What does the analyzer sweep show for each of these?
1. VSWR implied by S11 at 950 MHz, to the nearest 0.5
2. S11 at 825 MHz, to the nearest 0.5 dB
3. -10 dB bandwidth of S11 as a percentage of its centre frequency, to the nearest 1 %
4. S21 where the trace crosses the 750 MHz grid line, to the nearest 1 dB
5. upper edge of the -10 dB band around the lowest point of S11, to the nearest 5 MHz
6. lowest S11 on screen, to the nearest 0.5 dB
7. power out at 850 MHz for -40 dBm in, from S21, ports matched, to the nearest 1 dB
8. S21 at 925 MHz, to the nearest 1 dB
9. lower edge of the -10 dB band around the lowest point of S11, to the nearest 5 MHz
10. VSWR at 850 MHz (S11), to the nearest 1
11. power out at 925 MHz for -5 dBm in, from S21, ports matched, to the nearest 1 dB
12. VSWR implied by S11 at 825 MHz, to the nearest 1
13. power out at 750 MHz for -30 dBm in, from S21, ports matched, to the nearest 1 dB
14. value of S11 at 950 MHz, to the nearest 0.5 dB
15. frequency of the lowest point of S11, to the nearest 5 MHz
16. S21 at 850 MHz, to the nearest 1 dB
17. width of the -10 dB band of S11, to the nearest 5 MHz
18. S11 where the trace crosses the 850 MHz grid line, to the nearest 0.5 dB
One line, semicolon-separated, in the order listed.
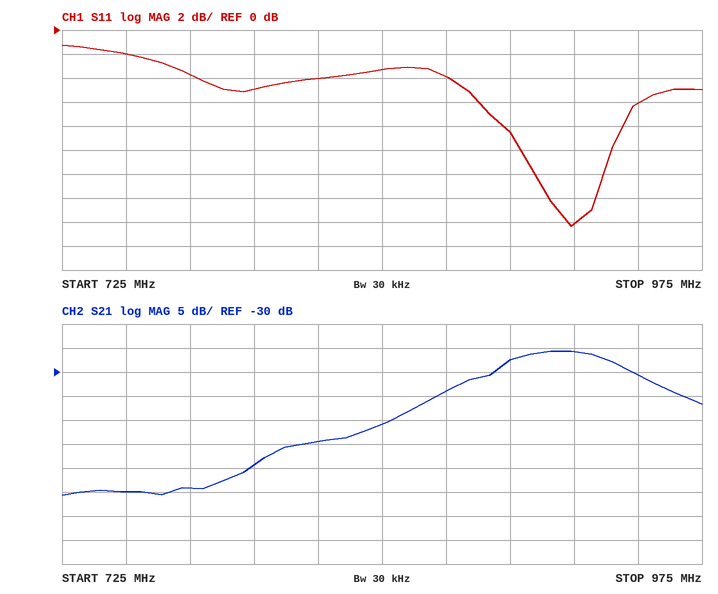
3.0; -4.0 dB; 4 %; -55 dB; 940 MHz; -16.5 dB; -81 dBm; -26 dB; 905 MHz; 5; -31 dBm; 4; -85 dBm; -6.0 dB; 925 MHz; -41 dB; 35 MHz; -3.5 dB
